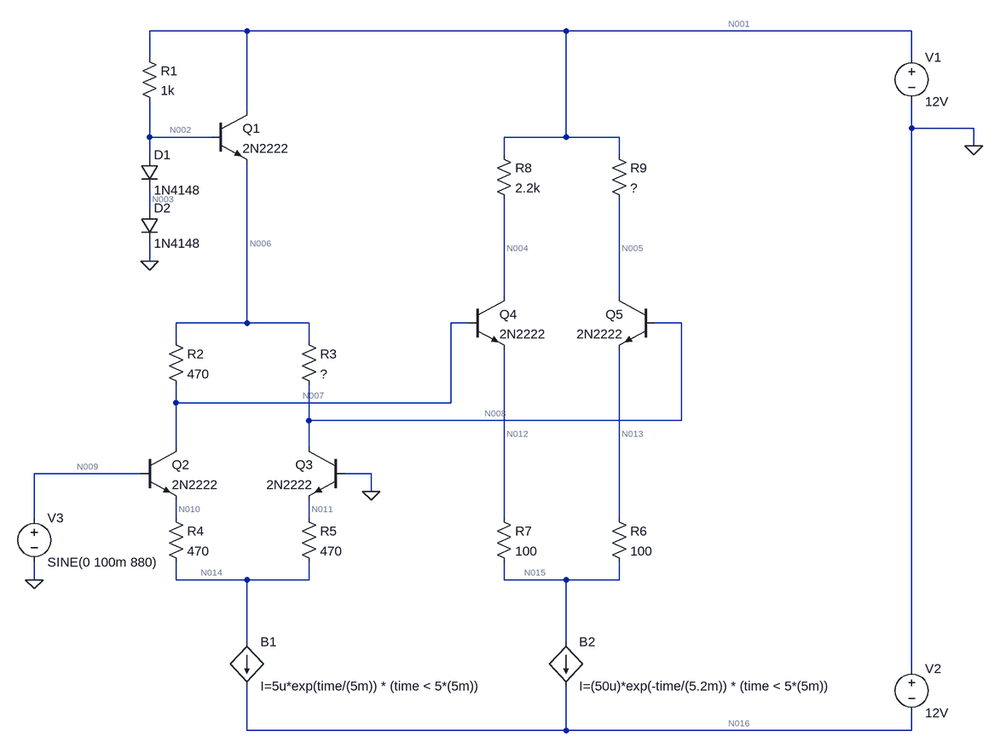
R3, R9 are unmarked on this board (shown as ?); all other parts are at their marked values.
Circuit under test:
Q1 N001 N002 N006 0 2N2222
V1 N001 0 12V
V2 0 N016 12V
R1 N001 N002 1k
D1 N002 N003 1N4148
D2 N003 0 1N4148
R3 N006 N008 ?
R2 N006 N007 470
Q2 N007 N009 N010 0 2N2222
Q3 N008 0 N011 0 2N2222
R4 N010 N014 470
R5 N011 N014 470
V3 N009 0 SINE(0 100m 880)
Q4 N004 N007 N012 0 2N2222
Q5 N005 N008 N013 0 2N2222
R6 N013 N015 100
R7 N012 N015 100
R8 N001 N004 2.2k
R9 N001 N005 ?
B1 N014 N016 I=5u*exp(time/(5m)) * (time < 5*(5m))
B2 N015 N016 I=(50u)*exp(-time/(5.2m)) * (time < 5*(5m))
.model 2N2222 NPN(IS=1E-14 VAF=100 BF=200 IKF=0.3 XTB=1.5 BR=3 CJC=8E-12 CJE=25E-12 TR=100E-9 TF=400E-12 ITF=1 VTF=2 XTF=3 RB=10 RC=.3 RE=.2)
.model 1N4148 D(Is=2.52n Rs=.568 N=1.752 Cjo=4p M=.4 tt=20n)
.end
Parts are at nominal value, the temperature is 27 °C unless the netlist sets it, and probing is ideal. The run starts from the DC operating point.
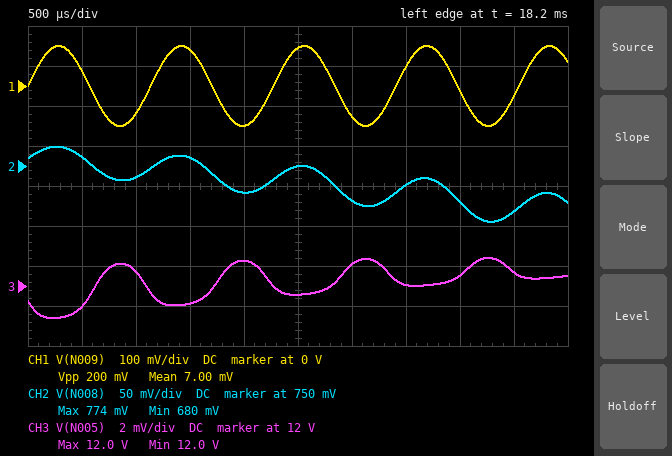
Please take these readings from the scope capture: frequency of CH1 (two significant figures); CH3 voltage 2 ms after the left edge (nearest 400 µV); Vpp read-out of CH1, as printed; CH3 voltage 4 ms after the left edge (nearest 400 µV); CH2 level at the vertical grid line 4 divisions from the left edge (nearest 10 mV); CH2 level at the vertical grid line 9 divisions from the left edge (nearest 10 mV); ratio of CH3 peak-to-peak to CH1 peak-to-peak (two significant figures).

880 Hz
11.9992 V
200 mV
11.9984 V
720 mV
690 mV
0.015
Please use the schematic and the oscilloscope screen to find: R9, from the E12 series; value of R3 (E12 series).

2.7 kΩ
270 Ω
